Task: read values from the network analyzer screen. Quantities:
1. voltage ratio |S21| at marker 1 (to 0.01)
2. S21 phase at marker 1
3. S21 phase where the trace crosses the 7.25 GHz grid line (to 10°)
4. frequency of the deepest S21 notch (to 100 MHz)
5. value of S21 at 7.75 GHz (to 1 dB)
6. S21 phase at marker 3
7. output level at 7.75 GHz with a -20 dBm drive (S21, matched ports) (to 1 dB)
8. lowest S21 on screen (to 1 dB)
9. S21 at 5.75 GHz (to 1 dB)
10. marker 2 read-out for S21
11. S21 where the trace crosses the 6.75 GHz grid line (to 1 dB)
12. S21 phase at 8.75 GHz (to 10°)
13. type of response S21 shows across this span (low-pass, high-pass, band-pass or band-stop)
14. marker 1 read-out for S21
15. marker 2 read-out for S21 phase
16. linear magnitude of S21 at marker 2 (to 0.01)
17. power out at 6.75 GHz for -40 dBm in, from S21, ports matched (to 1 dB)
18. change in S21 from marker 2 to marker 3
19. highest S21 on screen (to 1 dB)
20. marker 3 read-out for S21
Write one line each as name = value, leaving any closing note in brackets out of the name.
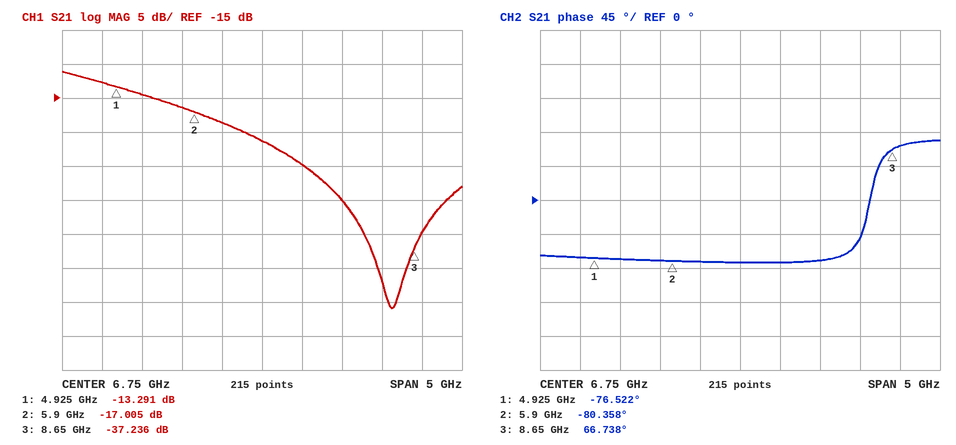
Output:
voltage ratio |S21| at marker 1 = 0.22
S21 phase at marker 1 = -76.522°
S21 phase where the trace crosses the 7.25 GHz grid line = -80°
frequency of the deepest S21 notch = 8.4 GHz
value of S21 at 7.75 GHz = -30 dB
S21 phase at marker 3 = 66.738°
output level at 7.75 GHz with a -20 dBm drive (S21, matched ports) = -50 dBm
lowest S21 on screen = -46 dB
S21 at 5.75 GHz = -16 dB
marker 2 read-out for S21 = -17.005 dB
S21 where the trace crosses the 6.75 GHz grid line = -21 dB
S21 phase at 8.75 GHz = 70°
type of response S21 shows across this span = low-pass
marker 1 read-out for S21 = -13.291 dB
marker 2 read-out for S21 phase = -80.358°
linear magnitude of S21 at marker 2 = 0.14
power out at 6.75 GHz for -40 dBm in, from S21, ports matched = -61 dBm
change in S21 from marker 2 to marker 3 = -20.231 dB
highest S21 on screen = -11 dB
marker 3 read-out for S21 = -37.236 dB
